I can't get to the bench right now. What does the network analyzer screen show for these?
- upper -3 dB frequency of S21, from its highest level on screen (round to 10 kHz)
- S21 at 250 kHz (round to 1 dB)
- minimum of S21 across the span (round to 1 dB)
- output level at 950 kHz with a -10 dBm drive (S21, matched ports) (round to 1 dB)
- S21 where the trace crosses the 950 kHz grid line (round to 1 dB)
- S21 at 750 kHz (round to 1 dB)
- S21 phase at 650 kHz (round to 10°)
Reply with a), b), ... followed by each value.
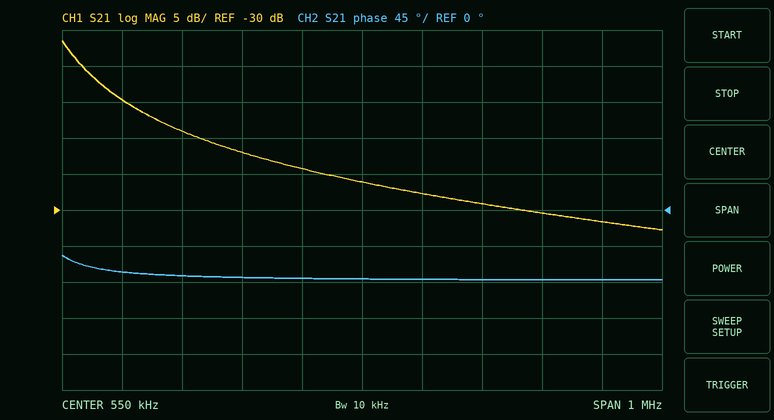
a) 80 kHz
b) -19 dB
c) -33 dB
d) -42 dBm
e) -32 dB
f) -29 dB
g) -90°
